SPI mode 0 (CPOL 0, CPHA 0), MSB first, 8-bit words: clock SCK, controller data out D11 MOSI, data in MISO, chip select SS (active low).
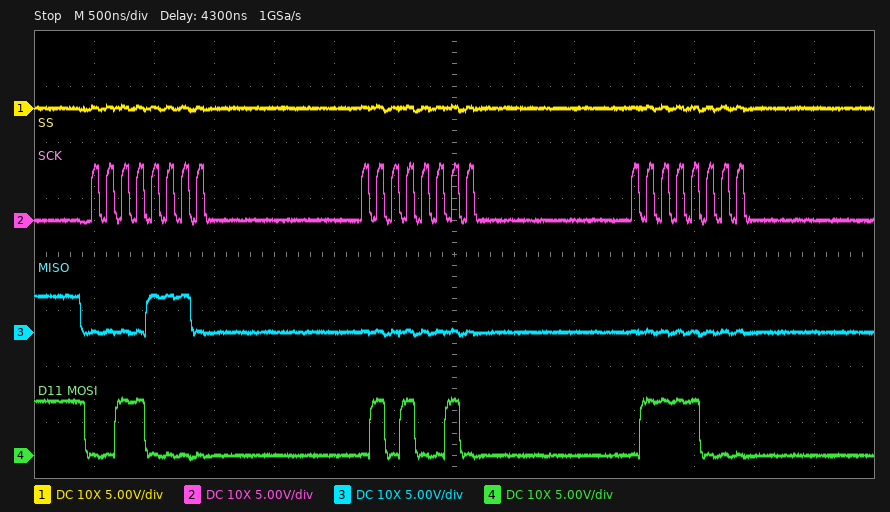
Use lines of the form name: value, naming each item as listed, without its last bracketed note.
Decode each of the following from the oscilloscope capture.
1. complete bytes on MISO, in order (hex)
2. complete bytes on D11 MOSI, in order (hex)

complete bytes on MISO, in order: 0E 00 00
complete bytes on D11 MOSI, in order: 30 52 78
